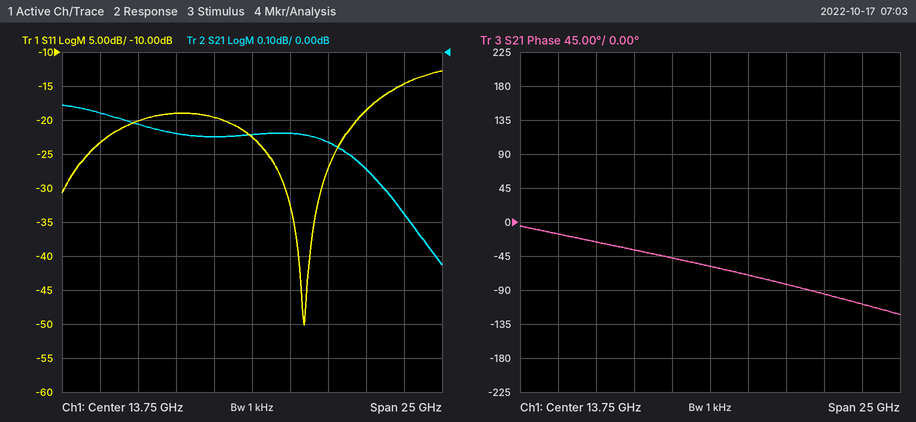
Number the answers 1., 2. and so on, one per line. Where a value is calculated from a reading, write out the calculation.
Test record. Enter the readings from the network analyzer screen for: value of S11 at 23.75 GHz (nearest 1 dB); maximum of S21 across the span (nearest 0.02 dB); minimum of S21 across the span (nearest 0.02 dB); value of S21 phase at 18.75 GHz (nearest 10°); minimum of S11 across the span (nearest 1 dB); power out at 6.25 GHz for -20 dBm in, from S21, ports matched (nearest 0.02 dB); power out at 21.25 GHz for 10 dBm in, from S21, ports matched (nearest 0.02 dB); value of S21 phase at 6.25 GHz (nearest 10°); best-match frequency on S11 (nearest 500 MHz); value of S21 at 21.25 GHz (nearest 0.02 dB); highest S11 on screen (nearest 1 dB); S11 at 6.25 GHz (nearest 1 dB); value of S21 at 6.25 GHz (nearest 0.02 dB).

1. -15 dB
2. -0.16 dB
3. -0.62 dB
4. -80°
5. -50 dB
6. -20 dBm + (-0.22 dB) = -20.22 dBm
7. 10 dBm + (-0.34 dB) = 9.66 dBm
8. -30°
9. 17.0 GHz
10. -0.34 dB
11. -13 dB
12. -20 dB
13. -0.22 dB
